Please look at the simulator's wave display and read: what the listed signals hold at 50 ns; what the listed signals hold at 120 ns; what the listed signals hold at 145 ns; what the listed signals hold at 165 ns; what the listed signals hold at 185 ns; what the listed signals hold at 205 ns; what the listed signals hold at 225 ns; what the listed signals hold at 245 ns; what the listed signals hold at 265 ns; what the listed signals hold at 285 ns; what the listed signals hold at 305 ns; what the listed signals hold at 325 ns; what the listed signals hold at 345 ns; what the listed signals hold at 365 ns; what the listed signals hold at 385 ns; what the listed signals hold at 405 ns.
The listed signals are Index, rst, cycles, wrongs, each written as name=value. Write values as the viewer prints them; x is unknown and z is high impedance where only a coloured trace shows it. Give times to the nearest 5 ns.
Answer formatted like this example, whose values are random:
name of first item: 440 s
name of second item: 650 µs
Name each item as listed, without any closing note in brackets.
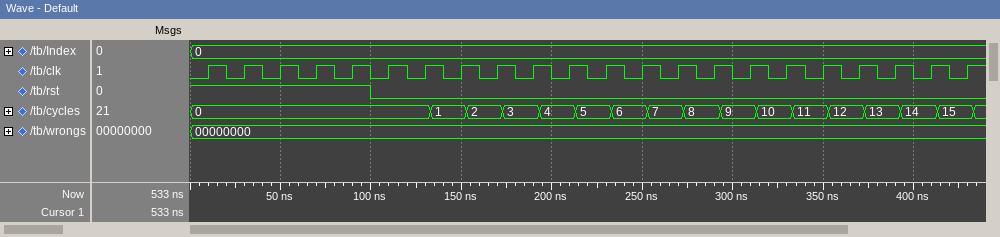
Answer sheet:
what the listed signals hold at 50 ns: Index=0, rst=1, cycles=0, wrongs=00000000
what the listed signals hold at 120 ns: Index=0, rst=0, cycles=0, wrongs=00000000
what the listed signals hold at 145 ns: Index=0, rst=0, cycles=1, wrongs=00000000
what the listed signals hold at 165 ns: Index=0, rst=0, cycles=2, wrongs=00000000
what the listed signals hold at 185 ns: Index=0, rst=0, cycles=3, wrongs=00000000
what the listed signals hold at 205 ns: Index=0, rst=0, cycles=4, wrongs=00000000
what the listed signals hold at 225 ns: Index=0, rst=0, cycles=5, wrongs=00000000
what the listed signals hold at 245 ns: Index=0, rst=0, cycles=6, wrongs=00000000
what the listed signals hold at 265 ns: Index=0, rst=0, cycles=7, wrongs=00000000
what the listed signals hold at 285 ns: Index=0, rst=0, cycles=8, wrongs=00000000
what the listed signals hold at 305 ns: Index=0, rst=0, cycles=9, wrongs=00000000
what the listed signals hold at 325 ns: Index=0, rst=0, cycles=10, wrongs=00000000
what the listed signals hold at 345 ns: Index=0, rst=0, cycles=11, wrongs=00000000
what the listed signals hold at 365 ns: Index=0, rst=0, cycles=12, wrongs=00000000
what the listed signals hold at 385 ns: Index=0, rst=0, cycles=13, wrongs=00000000
what the listed signals hold at 405 ns: Index=0, rst=0, cycles=14, wrongs=00000000
